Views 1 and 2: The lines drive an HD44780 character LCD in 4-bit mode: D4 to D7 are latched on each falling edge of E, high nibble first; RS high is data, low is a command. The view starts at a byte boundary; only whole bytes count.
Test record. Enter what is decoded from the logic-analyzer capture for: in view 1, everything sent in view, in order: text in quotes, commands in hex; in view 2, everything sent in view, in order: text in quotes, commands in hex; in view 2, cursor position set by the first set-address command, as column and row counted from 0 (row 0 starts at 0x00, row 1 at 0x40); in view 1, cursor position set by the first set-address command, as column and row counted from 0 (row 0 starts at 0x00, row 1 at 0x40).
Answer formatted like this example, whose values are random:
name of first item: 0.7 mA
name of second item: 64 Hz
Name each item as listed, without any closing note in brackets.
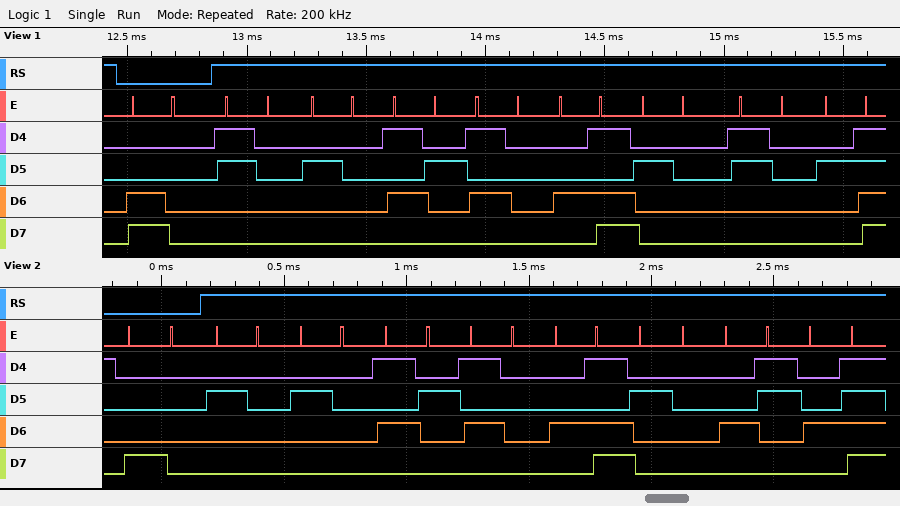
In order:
in view 1, everything sent in view, in order: text in quotes, commands in hex: 0xC0 "0 RPM 0/"
in view 2, everything sent in view, in order: text in quotes, commands in hex: 0x80 "  RPM CO"
in view 2, cursor position set by the first set-address command, as column and row counted from 0: column 0, row 0
in view 1, cursor position set by the first set-address command, as column and row counted from 0: column 0, row 1
